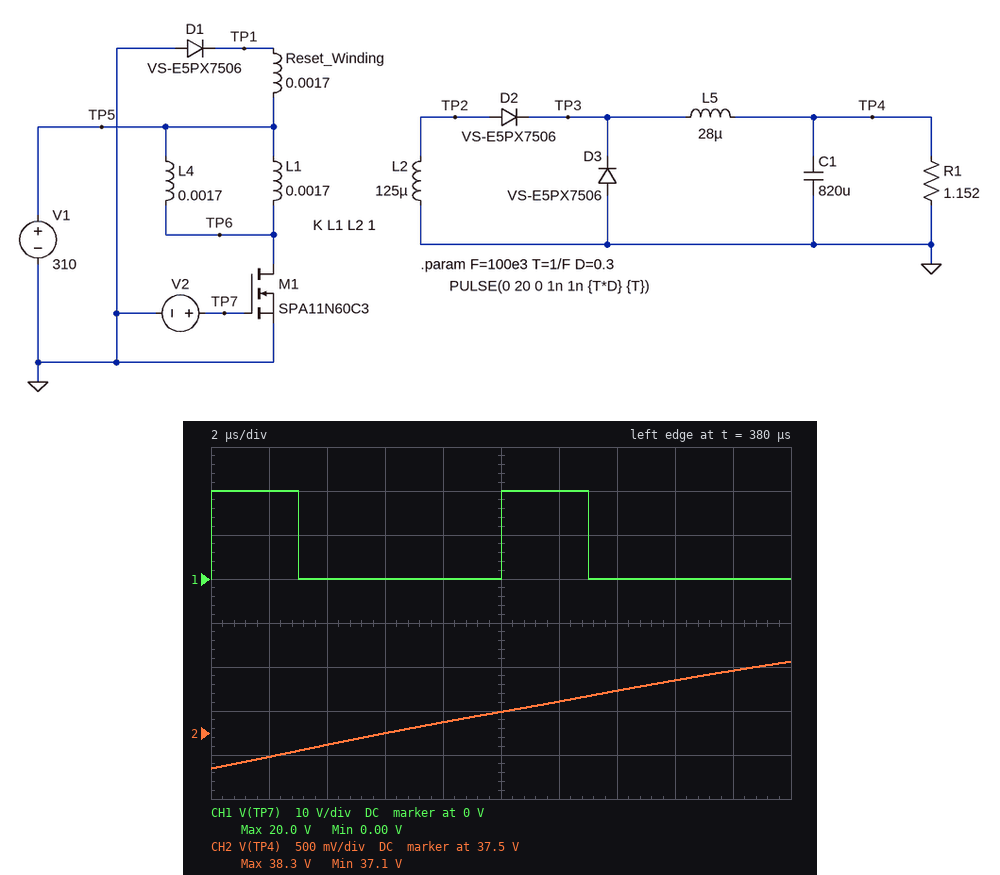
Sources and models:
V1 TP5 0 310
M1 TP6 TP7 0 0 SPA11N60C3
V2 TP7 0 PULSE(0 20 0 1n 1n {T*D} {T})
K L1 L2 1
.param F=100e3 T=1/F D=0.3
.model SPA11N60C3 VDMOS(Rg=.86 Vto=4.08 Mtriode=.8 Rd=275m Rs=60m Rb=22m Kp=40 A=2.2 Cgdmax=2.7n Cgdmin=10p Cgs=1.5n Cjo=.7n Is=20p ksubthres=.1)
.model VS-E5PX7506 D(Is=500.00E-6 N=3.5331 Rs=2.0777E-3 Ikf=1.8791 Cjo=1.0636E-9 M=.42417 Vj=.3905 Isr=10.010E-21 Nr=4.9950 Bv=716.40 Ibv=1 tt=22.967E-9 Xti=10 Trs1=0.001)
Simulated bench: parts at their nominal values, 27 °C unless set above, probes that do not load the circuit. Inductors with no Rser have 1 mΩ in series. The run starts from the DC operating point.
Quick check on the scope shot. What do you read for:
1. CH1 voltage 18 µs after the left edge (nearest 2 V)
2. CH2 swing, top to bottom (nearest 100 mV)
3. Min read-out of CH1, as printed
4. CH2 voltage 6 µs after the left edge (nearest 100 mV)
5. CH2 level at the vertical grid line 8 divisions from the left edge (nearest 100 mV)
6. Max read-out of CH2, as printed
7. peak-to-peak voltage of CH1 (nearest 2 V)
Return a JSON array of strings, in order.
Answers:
["0 V", "1.2 V", "0.00 V", "37.5 V", "38.1 V", "38.3 V", "20 V"]
